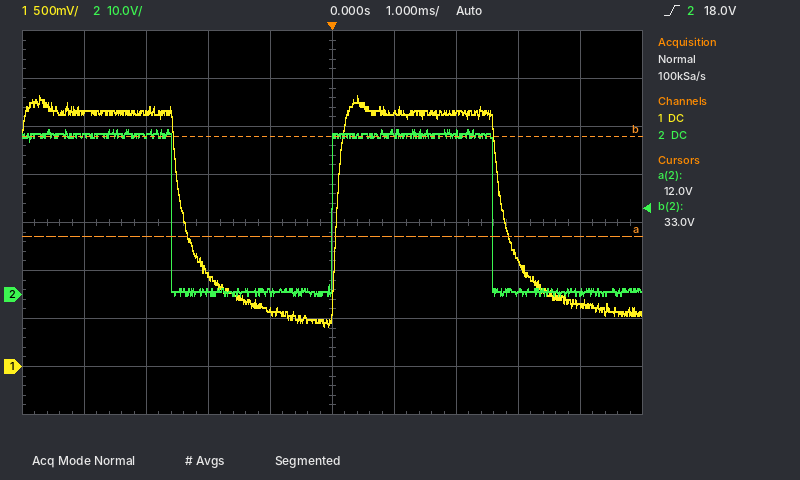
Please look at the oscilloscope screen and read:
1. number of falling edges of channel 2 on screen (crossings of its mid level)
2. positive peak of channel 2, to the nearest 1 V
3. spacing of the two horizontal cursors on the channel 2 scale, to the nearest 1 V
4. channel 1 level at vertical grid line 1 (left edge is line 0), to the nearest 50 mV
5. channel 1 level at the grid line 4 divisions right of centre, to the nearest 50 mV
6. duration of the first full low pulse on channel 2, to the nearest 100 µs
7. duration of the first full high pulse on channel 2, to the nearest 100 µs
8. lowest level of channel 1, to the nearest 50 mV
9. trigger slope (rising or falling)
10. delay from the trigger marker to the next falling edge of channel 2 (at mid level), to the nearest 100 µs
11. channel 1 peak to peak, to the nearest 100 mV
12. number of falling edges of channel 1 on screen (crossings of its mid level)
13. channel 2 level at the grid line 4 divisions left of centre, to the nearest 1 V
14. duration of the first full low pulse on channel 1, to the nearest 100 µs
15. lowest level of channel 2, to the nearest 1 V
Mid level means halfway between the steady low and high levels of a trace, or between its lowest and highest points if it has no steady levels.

2
34 V
21 V
2.65 V
650 mV
2.6 ms
2.6 ms
400 mV
rising
2.6 ms
2.40 V
2
33 V
2.5 ms
0 V
